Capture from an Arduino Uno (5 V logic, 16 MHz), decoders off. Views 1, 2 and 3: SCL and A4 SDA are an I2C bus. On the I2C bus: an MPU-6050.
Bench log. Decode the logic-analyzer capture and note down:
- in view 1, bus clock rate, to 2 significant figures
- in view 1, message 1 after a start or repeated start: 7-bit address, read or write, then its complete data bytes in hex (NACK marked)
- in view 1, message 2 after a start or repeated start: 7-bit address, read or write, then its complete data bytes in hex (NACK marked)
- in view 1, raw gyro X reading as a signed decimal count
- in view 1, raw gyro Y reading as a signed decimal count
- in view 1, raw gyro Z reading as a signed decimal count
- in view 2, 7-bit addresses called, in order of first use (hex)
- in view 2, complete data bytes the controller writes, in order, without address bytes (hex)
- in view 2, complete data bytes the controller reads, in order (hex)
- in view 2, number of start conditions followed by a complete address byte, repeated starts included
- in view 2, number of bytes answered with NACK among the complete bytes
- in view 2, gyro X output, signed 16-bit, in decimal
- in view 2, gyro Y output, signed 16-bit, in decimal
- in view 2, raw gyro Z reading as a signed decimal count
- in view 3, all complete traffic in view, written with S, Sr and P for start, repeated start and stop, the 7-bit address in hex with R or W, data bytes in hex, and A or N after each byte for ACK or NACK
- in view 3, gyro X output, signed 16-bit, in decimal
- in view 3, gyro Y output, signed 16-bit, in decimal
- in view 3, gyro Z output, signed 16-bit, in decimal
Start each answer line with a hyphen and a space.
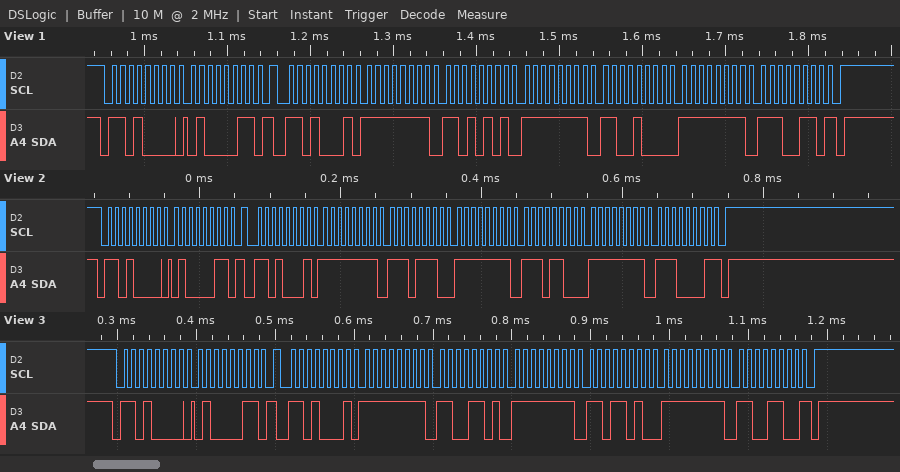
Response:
- 100 kHz
- 0x68 write: 43
- 0x68 read: FF D5 FF C8 FF E6 NACK
- -43
- -56
- -26
- 0x68
- 43
- FF EE FF EC FF E1
- 2
- 1
- -18
- -20
- -31
- S 68W A 43 A Sr 68R A FF A CD A FF A DA A FF A CC N P
- -51
- -38
- -52
